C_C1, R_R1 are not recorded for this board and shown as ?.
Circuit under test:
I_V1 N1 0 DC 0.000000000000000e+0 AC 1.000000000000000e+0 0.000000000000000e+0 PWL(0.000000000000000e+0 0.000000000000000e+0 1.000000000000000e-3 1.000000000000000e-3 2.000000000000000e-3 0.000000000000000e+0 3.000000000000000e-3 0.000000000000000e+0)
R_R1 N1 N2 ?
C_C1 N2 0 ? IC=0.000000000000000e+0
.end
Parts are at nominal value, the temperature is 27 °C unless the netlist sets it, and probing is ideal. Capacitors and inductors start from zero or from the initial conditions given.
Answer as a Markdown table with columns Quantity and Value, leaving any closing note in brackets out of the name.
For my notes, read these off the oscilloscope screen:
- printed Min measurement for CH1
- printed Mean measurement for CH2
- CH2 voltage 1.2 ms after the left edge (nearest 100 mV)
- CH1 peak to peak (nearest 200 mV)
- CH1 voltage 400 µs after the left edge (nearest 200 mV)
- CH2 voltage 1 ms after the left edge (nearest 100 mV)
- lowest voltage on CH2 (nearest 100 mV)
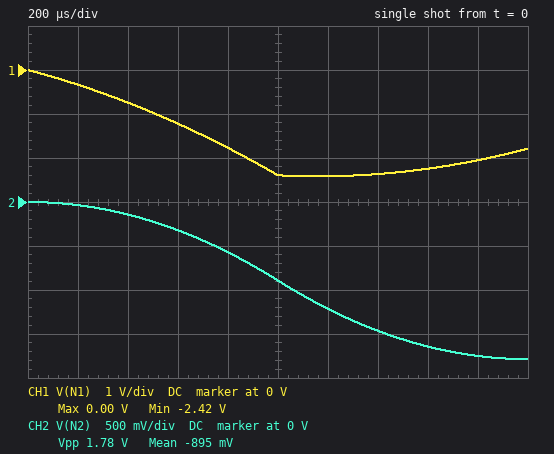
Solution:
| Quantity | Value |
|---|---|
| printed Min measurement for CH1 | -2.42 V |
| printed Mean measurement for CH2 | -895 mV |
| CH2 voltage 1.2 ms after the left edge | -1.2 V |
| CH1 peak to peak | 2.4 V |
| CH1 voltage 400 µs after the left edge | -800 mV |
| CH2 voltage 1 ms after the left edge | -900 mV |
| lowest voltage on CH2 | -1.8 V |
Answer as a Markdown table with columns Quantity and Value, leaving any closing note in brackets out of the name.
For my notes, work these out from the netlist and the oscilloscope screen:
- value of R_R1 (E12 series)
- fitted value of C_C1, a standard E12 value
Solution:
| Quantity | Value |
|---|---|
| value of R_R1 | 1.5 kΩ |
| fitted value of C_C1, a standard E12 value | 560 nF |
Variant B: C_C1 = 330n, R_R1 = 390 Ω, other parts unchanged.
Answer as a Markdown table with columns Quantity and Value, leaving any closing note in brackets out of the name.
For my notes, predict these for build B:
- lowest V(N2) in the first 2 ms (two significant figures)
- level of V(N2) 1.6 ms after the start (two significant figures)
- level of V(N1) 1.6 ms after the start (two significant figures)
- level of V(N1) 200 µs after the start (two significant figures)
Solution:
| Quantity | Value |
|---|---|
| lowest V(N2) in the first 2 ms | -3.0 V |
| level of V(N2) 1.6 ms after the start | -2.8 V |
| level of V(N1) 1.6 ms after the start | -2.9 V |
| level of V(N1) 200 µs after the start | -140 mV |
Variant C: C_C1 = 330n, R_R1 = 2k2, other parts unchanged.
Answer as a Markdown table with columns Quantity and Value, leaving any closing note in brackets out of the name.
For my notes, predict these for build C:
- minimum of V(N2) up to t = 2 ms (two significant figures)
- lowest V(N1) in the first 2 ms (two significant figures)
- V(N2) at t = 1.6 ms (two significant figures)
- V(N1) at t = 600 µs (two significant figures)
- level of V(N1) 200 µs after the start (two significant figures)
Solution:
| Quantity | Value |
|---|---|
| minimum of V(N2) up to t = 2 ms | -3.0 V |
| lowest V(N1) in the first 2 ms | -3.8 V |
| V(N2) at t = 1.6 ms | -2.8 V |
| V(N1) at t = 600 µs | -1.9 V |
| level of V(N1) 200 µs after the start | -500 mV |
